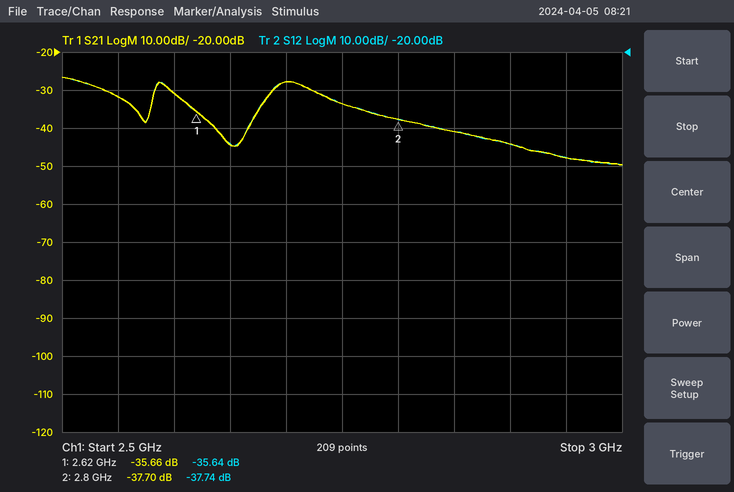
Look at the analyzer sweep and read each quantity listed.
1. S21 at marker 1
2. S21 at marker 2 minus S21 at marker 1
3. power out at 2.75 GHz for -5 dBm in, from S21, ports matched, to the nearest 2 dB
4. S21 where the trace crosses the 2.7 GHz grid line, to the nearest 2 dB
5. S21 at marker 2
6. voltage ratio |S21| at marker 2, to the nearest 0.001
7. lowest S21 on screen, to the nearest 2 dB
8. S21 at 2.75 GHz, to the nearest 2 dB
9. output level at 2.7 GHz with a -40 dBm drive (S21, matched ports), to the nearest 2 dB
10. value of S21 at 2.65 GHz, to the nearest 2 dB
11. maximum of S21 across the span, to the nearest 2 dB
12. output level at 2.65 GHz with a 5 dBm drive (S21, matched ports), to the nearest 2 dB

-35.66 dB
-2.04 dB
-38 dBm
-28 dB
-37.70 dB
0.013
-50 dB
-34 dB
-68 dBm
-44 dB
-26 dB
-40 dBm
